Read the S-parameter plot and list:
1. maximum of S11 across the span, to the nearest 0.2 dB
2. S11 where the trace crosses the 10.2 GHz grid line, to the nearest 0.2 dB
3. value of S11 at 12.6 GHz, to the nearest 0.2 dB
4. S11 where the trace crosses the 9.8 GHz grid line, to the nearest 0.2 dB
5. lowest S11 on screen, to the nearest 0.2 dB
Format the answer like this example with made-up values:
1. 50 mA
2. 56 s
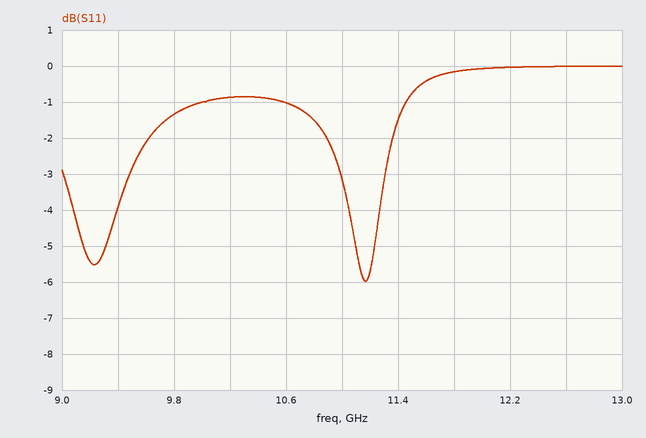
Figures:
1. 0.0 dB
2. -0.8 dB
3. 0.0 dB
4. -1.4 dB
5. -6.0 dB
